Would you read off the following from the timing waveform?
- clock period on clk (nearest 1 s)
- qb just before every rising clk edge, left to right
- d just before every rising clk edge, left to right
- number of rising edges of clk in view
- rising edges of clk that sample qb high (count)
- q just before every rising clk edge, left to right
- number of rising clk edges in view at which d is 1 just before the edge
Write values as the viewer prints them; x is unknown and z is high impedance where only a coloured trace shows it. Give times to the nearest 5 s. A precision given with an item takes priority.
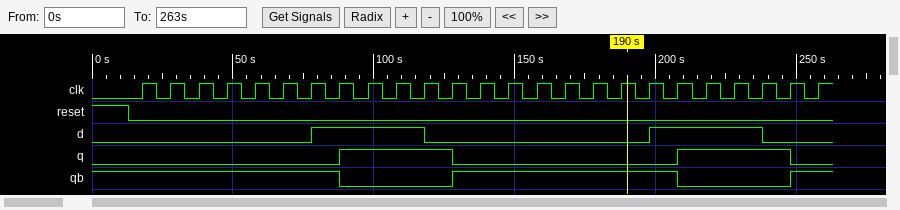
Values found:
10 s
1 1 1 1 1 1 1 1 0 0 0 0 1 1 1 1 1 1 1 1 0 0 0 0 1
0 0 0 0 0 0 0 1 1 1 1 0 0 0 0 0 0 0 0 1 1 1 1 0 0
25
17
0 0 0 0 0 0 0 0 1 1 1 1 0 0 0 0 0 0 0 0 1 1 1 1 0
8
